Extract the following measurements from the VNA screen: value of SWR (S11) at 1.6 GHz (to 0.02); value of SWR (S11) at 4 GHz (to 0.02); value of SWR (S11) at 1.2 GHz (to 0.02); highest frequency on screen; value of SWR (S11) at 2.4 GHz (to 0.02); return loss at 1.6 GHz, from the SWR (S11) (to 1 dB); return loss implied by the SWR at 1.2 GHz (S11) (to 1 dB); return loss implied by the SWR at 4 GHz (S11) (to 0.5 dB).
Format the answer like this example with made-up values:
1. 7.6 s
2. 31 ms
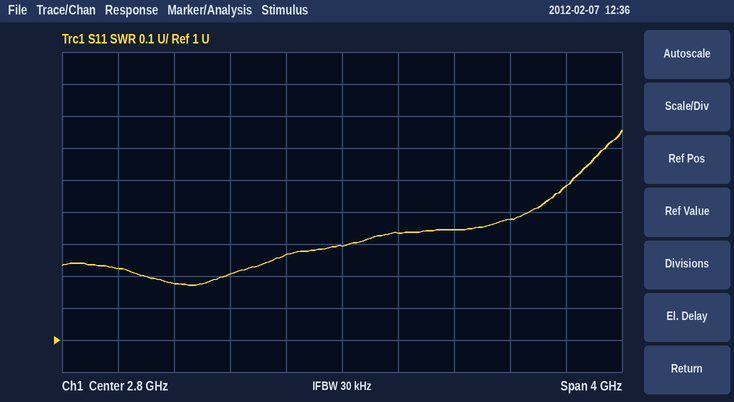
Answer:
1. 1.18
2. 1.38
3. 1.22
4. 4.8 GHz
5. 1.26
6. 22 dB
7. 20 dB
8. 16.0 dB
